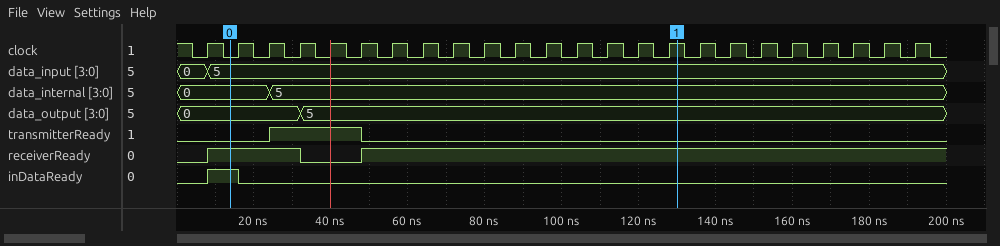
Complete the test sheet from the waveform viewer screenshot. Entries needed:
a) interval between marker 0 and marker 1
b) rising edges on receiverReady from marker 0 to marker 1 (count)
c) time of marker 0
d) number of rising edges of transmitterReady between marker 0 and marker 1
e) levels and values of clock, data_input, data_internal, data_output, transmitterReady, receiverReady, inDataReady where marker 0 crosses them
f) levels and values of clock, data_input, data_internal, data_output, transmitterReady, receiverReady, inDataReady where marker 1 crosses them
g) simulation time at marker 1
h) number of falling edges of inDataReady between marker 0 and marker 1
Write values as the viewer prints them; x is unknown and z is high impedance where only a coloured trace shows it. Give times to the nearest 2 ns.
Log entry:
116 ns
1
14 ns
1
clock=0, data_input=5, data_internal=0, data_output=0, transmitterReady=0, receiverReady=1, inDataReady=1
clock=1, data_input=5, data_internal=5, data_output=5, transmitterReady=0, receiverReady=1, inDataReady=0
130 ns
1
